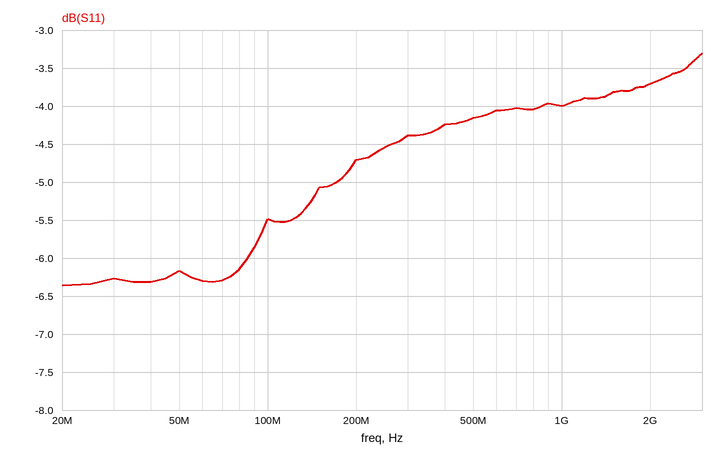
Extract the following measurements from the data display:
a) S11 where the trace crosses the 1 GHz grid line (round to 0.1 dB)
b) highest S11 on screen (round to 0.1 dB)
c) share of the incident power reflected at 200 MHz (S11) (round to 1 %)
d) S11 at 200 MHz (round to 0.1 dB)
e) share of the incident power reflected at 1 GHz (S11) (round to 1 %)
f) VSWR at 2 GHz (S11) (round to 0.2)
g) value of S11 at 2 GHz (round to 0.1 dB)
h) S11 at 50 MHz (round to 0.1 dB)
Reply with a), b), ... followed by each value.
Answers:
a) -4.0 dB
b) -3.3 dB
c) 34 %
d) -4.7 dB
e) 40 %
f) 4.8
g) -3.7 dB
h) -6.2 dB
